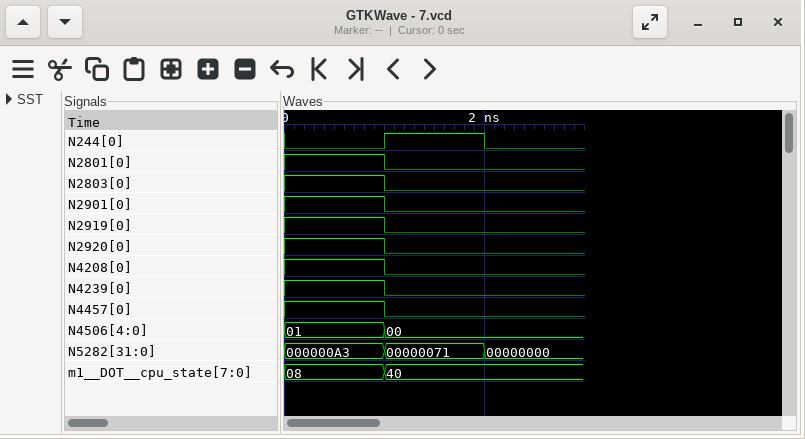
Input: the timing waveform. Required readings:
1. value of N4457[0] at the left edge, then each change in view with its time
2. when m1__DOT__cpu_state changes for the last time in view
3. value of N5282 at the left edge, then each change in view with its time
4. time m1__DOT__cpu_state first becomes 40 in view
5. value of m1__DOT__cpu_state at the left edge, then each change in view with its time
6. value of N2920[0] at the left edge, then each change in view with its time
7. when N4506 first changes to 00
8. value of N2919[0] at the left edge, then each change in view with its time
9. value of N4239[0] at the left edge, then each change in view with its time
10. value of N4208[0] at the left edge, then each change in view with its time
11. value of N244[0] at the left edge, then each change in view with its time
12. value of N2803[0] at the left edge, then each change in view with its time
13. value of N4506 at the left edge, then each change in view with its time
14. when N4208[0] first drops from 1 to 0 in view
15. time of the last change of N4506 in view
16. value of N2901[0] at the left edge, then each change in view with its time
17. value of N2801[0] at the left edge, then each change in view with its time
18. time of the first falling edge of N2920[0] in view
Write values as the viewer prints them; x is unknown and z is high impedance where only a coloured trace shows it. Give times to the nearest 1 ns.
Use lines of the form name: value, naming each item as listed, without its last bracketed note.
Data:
value of N4457[0] at the left edge, then each change in view with its time: 1, 0 at 1 ns
when m1__DOT__cpu_state changes for the last time in view: 1 ns
value of N5282 at the left edge, then each change in view with its time: 000000A3, 00000071 at 1 ns, 00000000 at 2 ns
time m1__DOT__cpu_state first becomes 40 in view: 1 ns
value of m1__DOT__cpu_state at the left edge, then each change in view with its time: 08, 40 at 1 ns
value of N2920[0] at the left edge, then each change in view with its time: 1, 0 at 1 ns
when N4506 first changes to 00: 1 ns
value of N2919[0] at the left edge, then each change in view with its time: 1, 0 at 1 ns
value of N4239[0] at the left edge, then each change in view with its time: 1, 0 at 1 ns
value of N4208[0] at the left edge, then each change in view with its time: 1, 0 at 1 ns
value of N244[0] at the left edge, then each change in view with its time: 0, 1 at 1 ns, 0 at 2 ns
value of N2803[0] at the left edge, then each change in view with its time: 1, 0 at 1 ns
value of N4506 at the left edge, then each change in view with its time: 01, 00 at 1 ns
when N4208[0] first drops from 1 to 0 in view: 1 ns
time of the last change of N4506 in view: 1 ns
value of N2901[0] at the left edge, then each change in view with its time: 1, 0 at 1 ns
value of N2801[0] at the left edge, then each change in view with its time: 1, 0 at 1 ns
time of the first falling edge of N2920[0] in view: 1 ns
